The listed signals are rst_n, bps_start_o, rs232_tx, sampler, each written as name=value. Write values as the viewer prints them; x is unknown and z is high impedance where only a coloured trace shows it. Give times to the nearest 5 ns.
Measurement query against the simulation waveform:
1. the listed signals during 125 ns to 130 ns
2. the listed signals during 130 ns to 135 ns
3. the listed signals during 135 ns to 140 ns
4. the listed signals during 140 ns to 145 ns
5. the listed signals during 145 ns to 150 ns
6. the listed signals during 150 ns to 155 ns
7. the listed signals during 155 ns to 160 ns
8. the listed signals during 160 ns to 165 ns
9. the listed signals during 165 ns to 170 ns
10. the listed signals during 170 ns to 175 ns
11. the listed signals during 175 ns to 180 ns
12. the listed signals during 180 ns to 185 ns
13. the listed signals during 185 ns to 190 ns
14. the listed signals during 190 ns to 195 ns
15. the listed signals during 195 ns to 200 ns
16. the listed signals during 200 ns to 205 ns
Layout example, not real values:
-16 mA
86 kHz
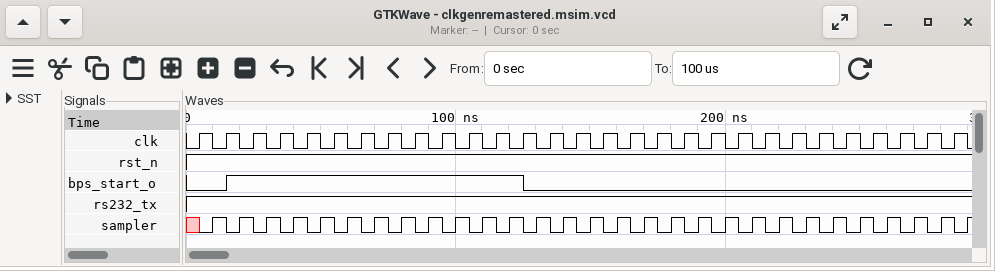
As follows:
rst_n=1, bps_start_o=0, rs232_tx=1, sampler=0
rst_n=1, bps_start_o=0, rs232_tx=1, sampler=1
rst_n=1, bps_start_o=0, rs232_tx=1, sampler=0
rst_n=1, bps_start_o=0, rs232_tx=1, sampler=1
rst_n=1, bps_start_o=0, rs232_tx=1, sampler=0
rst_n=1, bps_start_o=0, rs232_tx=1, sampler=1
rst_n=1, bps_start_o=0, rs232_tx=1, sampler=0
rst_n=1, bps_start_o=0, rs232_tx=1, sampler=1
rst_n=1, bps_start_o=0, rs232_tx=1, sampler=0
rst_n=1, bps_start_o=0, rs232_tx=1, sampler=1
rst_n=1, bps_start_o=0, rs232_tx=1, sampler=0
rst_n=1, bps_start_o=0, rs232_tx=1, sampler=1
rst_n=1, bps_start_o=0, rs232_tx=1, sampler=0
rst_n=1, bps_start_o=0, rs232_tx=1, sampler=1
rst_n=1, bps_start_o=0, rs232_tx=1, sampler=0
rst_n=1, bps_start_o=0, rs232_tx=1, sampler=1
